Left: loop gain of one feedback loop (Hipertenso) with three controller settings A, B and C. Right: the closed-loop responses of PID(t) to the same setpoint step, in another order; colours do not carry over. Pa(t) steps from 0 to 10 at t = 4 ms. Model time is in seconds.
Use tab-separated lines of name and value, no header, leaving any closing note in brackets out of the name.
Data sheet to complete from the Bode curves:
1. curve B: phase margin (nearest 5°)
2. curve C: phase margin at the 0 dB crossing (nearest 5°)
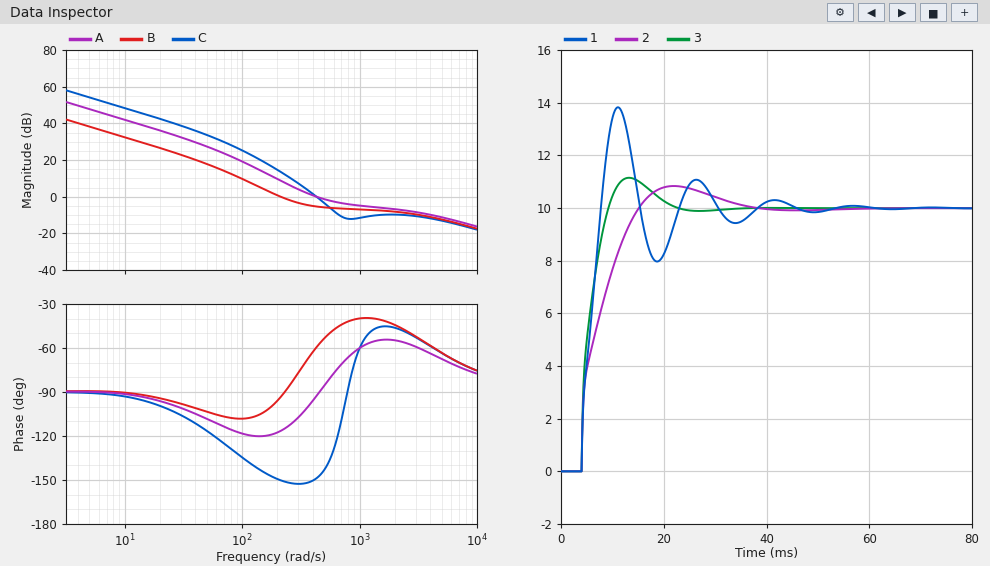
curve B: phase margin	85°
curve C: phase margin at the 0 dB crossing	30°
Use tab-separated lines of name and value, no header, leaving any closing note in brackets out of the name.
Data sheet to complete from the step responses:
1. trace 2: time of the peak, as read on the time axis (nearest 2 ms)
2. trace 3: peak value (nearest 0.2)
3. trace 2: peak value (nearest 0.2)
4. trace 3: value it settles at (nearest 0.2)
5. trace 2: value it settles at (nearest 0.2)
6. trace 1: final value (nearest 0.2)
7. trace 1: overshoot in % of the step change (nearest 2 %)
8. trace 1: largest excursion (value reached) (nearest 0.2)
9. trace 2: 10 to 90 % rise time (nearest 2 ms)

trace 2: time of the peak, as read on the time axis	22 ms
trace 3: peak value	11.2
trace 2: peak value	10.8
trace 3: value it settles at	10.0
trace 2: value it settles at	10.0
trace 1: final value	10.0
trace 1: overshoot in % of the step change	38 %
trace 1: largest excursion (value reached)	13.8
trace 2: 10 to 90 % rise time	8 ms
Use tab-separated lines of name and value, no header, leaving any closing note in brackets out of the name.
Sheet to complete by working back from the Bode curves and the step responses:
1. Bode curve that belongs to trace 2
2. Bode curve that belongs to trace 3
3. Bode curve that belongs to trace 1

Bode curve that belongs to trace 2	B
Bode curve that belongs to trace 3	A
Bode curve that belongs to trace 1	C
